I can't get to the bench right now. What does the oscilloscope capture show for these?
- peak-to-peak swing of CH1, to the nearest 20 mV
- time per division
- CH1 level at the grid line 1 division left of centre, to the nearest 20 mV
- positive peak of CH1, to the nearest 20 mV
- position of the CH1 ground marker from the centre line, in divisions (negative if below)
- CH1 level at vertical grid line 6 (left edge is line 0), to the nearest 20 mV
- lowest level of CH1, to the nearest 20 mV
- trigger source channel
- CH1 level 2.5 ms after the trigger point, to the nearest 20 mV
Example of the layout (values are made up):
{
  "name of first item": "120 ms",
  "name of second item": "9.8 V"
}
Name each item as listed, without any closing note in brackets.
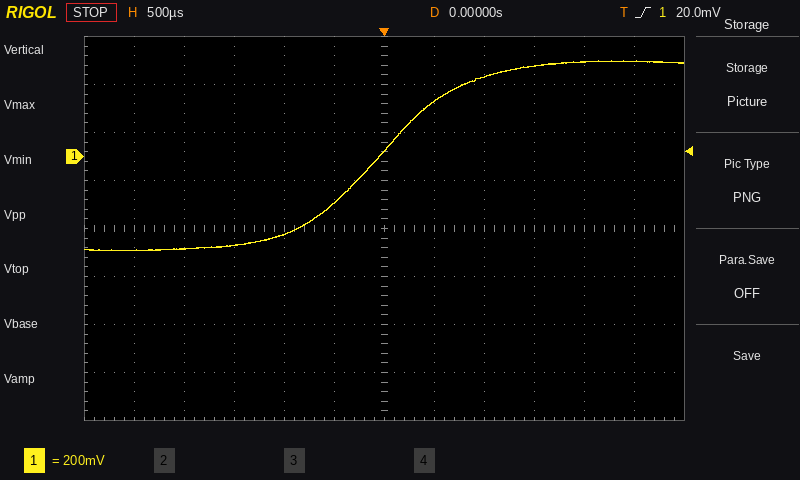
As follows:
{
  "peak-to-peak swing of CH1, to the nearest 20 mV": "800 mV",
  "time per division": "500 µs",
  "CH1 level at the grid line 1 division left of centre, to the nearest 20 mV": "-200 mV",
  "positive peak of CH1, to the nearest 20 mV": "400 mV",
  "position of the CH1 ground marker from the centre line, in divisions": "+1.5 div",
  "CH1 level at vertical grid line 6 (left edge is line 0), to the nearest 20 mV": "20 mV",
  "lowest level of CH1, to the nearest 20 mV": "-400 mV",
  "trigger source channel": "CH1",
  "CH1 level 2.5 ms after the trigger point, to the nearest 20 mV": "400 mV"
}
